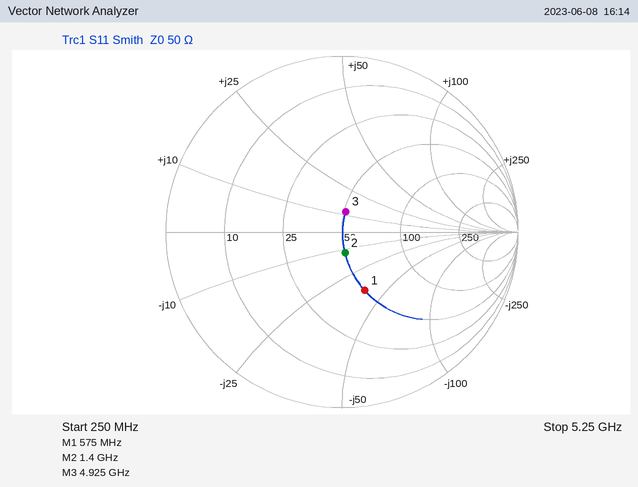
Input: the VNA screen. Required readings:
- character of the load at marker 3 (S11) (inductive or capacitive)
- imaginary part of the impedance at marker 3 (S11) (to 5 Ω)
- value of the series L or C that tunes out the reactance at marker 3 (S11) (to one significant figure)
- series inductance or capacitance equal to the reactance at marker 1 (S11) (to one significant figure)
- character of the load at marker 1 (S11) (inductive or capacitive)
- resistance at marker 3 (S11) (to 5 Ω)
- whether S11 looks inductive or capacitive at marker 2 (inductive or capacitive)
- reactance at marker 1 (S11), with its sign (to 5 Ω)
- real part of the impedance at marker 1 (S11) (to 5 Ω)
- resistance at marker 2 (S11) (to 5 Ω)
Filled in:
inductive
+10 Ω
3 pF
7 pF
capacitive
50 Ω
capacitive
-40 Ω
50 Ω
50 Ω
